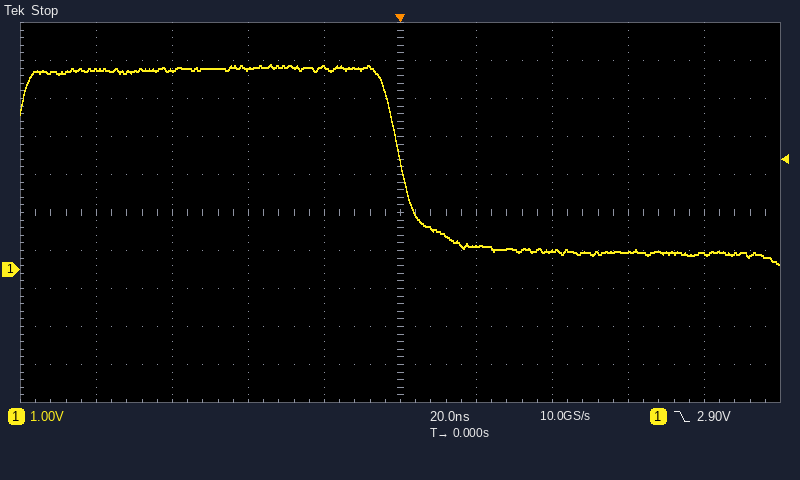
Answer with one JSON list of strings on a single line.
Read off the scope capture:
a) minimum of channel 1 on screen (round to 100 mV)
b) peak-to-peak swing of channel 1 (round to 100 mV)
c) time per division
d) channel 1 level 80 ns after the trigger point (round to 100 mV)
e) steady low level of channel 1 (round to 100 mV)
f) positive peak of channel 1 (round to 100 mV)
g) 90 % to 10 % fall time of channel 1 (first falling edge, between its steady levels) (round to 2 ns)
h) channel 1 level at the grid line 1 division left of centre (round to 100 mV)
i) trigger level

["100 mV", "5.3 V", "20 ns", "400 mV", "400 mV", "5.4 V", "16 ns", "5.3 V", "2.90 V"]
